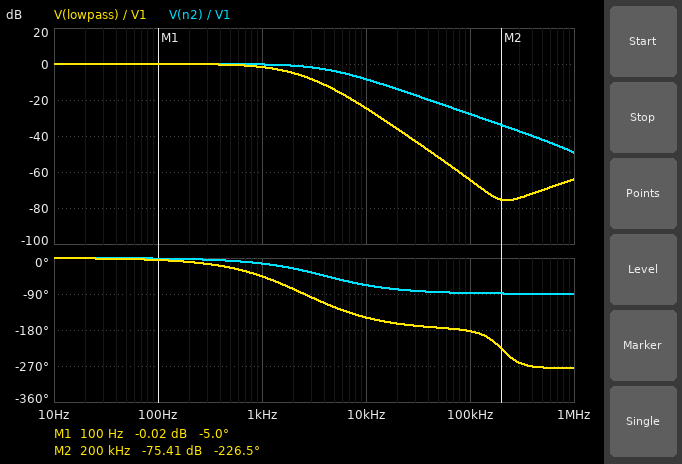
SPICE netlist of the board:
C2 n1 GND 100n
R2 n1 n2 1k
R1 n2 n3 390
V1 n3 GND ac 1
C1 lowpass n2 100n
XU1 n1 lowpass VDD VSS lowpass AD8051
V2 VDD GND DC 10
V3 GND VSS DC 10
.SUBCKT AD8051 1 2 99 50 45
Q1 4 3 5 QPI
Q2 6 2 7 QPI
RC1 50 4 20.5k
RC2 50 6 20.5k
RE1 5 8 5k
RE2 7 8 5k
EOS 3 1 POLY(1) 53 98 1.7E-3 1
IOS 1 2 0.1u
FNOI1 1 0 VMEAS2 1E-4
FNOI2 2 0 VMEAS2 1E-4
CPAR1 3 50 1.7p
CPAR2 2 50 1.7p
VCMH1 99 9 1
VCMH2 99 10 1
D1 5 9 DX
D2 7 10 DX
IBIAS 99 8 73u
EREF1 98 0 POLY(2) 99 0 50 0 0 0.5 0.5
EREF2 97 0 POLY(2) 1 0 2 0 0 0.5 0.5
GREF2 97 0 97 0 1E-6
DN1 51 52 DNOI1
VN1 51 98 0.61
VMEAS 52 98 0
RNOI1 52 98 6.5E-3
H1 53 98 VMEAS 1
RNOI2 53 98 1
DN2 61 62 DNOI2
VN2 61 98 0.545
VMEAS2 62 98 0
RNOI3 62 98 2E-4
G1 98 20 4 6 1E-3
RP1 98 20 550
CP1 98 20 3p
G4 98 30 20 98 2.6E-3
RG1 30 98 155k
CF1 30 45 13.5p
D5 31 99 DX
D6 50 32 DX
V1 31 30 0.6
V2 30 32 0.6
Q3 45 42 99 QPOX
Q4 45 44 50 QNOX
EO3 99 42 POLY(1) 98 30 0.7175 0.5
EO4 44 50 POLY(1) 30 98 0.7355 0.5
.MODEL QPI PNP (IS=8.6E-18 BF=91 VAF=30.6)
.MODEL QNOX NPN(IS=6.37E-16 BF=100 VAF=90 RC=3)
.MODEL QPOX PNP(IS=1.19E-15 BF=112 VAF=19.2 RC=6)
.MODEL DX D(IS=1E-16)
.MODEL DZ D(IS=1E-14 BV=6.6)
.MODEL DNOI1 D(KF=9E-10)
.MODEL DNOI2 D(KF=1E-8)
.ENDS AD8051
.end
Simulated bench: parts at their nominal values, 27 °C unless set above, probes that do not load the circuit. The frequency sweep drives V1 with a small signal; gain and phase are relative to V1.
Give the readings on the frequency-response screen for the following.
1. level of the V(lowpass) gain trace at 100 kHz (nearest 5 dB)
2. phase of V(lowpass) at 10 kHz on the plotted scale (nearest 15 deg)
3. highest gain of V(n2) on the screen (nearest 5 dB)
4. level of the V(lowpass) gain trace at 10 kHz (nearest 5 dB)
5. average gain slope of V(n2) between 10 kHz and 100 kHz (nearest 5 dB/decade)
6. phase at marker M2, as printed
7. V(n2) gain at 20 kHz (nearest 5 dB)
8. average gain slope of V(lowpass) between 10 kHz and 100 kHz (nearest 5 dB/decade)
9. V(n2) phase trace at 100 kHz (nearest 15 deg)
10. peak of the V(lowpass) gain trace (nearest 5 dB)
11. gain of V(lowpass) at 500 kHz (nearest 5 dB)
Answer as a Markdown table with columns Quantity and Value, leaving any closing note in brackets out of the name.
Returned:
| Quantity | Value |
|---|---|
| level of the V(lowpass) gain trace at 100 kHz | -65 dB |
| phase of V(lowpass) at 10 kHz on the plotted scale | -150 deg |
| highest gain of V(n2) on the screen | 0 dB |
| level of the V(lowpass) gain trace at 10 kHz | -25 dB |
| average gain slope of V(n2) between 10 kHz and 100 kHz | -20 dB/decade |
| phase at marker M2, as printed | -226.5 deg |
| V(n2) gain at 20 kHz | -15 dB |
| average gain slope of V(lowpass) between 10 kHz and 100 kHz | -40 dB/decade |
| V(n2) phase trace at 100 kHz | -90 deg |
| peak of the V(lowpass) gain trace | 0 dB |
| gain of V(lowpass) at 500 kHz | -70 dB |
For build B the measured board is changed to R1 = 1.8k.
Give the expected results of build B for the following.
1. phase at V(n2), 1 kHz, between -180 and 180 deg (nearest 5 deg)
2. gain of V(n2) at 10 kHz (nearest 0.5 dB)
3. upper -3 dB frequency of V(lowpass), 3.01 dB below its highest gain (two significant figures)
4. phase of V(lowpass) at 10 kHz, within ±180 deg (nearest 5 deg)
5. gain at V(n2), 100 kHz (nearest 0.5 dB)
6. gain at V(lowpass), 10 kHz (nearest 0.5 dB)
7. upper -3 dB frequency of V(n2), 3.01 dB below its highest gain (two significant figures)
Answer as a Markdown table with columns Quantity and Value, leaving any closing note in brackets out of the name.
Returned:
| Quantity | Value |
|---|---|
| phase at V(n2), 1 kHz, between -180 and 180 deg | -50 deg |
| gain of V(n2) at 10 kHz | -21.0 dB |
| upper -3 dB frequency of V(lowpass), 3.01 dB below its highest gain | 720 Hz |
| phase of V(lowpass) at 10 kHz, within ±180 deg | -165 deg |
| gain at V(n2), 100 kHz | -41.0 dB |
| gain at V(lowpass), 10 kHz | -37.0 dB |
| upper -3 dB frequency of V(n2), 3.01 dB below its highest gain | 880 Hz |
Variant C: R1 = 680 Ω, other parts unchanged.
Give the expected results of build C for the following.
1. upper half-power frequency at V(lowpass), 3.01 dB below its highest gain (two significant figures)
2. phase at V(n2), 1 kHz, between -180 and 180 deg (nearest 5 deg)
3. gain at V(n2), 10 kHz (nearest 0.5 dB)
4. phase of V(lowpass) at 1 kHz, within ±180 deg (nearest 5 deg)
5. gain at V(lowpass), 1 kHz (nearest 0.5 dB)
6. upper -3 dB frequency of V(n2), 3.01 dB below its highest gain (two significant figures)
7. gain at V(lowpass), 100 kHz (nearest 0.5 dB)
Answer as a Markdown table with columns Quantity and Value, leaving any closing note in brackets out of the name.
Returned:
| Quantity | Value |
|---|---|
| upper half-power frequency at V(lowpass), 3.01 dB below its highest gain | 1.2 kHz |
| phase at V(n2), 1 kHz, between -180 and 180 deg | -25 deg |
| gain at V(n2), 10 kHz | -13.0 dB |
| phase of V(lowpass) at 1 kHz, within ±180 deg | -55 deg |
| gain at V(lowpass), 1 kHz | -2.0 dB |
| upper -3 dB frequency of V(n2), 3.01 dB below its highest gain | 2.3 kHz |
| gain at V(lowpass), 100 kHz | -69.0 dB |
